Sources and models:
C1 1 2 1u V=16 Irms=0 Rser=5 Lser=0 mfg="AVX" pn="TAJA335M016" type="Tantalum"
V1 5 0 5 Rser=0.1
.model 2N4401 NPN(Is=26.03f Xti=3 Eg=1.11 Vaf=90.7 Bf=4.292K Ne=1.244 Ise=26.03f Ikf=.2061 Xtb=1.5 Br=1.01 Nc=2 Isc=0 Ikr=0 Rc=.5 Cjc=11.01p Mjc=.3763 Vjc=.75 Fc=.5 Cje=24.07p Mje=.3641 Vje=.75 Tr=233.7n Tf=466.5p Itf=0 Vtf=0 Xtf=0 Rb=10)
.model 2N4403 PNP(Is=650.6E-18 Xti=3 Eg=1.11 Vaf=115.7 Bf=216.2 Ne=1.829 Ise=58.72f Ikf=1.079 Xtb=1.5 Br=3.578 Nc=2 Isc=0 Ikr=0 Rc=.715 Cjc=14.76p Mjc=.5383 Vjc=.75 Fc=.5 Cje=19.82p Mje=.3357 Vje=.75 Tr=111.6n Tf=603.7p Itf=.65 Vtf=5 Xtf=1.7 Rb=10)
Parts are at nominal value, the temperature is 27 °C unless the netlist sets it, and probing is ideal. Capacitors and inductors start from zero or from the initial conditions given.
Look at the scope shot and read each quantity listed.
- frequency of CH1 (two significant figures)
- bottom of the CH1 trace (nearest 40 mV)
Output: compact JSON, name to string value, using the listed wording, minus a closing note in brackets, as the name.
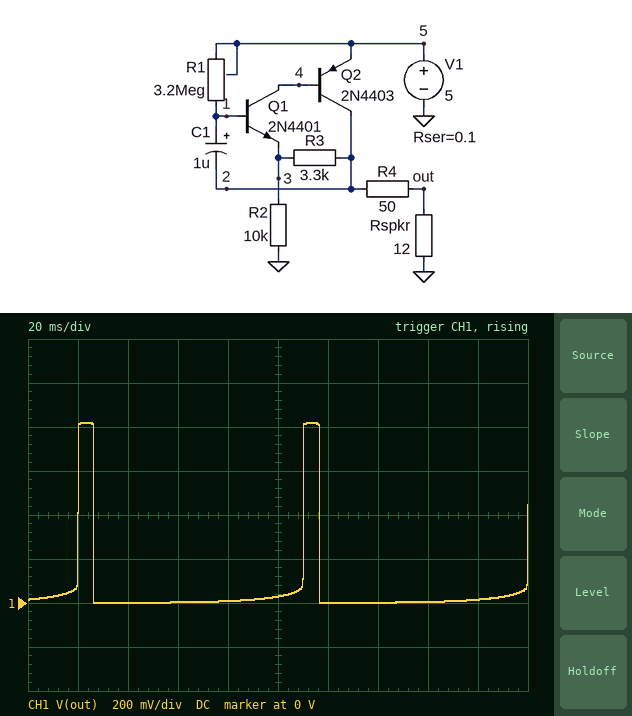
{"frequency of CH1": "11 Hz", "bottom of the CH1 trace": "0 V"}
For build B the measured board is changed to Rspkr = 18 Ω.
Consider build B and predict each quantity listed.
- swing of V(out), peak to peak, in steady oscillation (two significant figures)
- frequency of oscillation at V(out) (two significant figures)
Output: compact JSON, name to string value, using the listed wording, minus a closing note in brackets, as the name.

{"swing of V(out), peak to peak, in steady oscillation": "1.1 V", "frequency of oscillation at V(out)": "7.1 Hz"}
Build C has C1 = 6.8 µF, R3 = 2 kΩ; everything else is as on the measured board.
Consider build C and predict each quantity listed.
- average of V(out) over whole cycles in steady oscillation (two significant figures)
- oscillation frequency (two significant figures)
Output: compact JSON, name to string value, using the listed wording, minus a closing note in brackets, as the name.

{"average of V(out) over whole cycles in steady oscillation": "89 mV", "oscillation frequency": "2.8 Hz"}
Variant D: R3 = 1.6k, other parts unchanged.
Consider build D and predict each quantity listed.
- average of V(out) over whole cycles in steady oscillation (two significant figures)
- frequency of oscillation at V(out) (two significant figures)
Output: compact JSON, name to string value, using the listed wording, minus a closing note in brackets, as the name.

{"average of V(out) over whole cycles in steady oscillation": "110 mV", "frequency of oscillation at V(out)": "25 Hz"}
